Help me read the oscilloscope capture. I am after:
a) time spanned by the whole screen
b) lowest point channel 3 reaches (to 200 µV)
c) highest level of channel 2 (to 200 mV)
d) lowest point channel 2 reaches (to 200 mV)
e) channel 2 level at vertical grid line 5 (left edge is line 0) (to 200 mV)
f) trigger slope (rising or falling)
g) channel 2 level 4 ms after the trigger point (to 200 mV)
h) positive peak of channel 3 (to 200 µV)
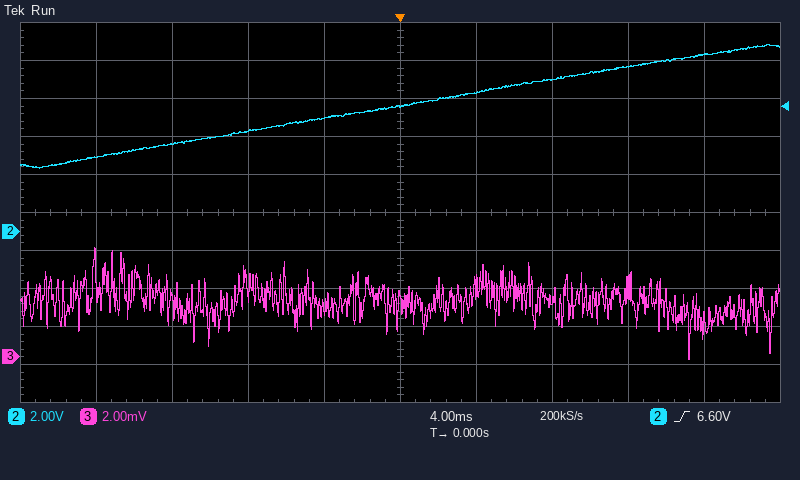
40 ms
-200 µV
9.8 V
3.4 V
6.6 V
rising
7.4 V
5.8 mV
